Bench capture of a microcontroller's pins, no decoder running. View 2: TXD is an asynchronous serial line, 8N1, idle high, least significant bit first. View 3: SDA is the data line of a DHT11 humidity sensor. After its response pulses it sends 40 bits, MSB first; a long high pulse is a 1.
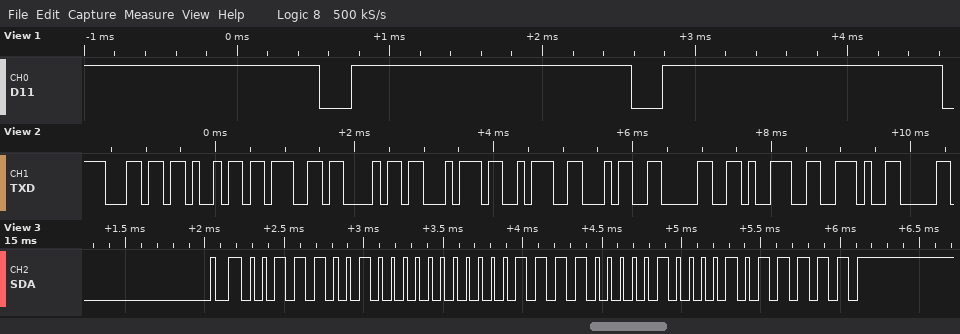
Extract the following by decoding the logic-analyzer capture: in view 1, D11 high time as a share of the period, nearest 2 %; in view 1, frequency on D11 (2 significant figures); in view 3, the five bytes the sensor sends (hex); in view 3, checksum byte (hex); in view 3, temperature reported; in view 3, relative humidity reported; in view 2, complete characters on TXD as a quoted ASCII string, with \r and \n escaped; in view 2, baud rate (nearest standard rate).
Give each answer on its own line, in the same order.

90 %
490 Hz
39 00 1E 08 5F
0x5F
30.8 °C
57 %
"light:409."
9600 baud
